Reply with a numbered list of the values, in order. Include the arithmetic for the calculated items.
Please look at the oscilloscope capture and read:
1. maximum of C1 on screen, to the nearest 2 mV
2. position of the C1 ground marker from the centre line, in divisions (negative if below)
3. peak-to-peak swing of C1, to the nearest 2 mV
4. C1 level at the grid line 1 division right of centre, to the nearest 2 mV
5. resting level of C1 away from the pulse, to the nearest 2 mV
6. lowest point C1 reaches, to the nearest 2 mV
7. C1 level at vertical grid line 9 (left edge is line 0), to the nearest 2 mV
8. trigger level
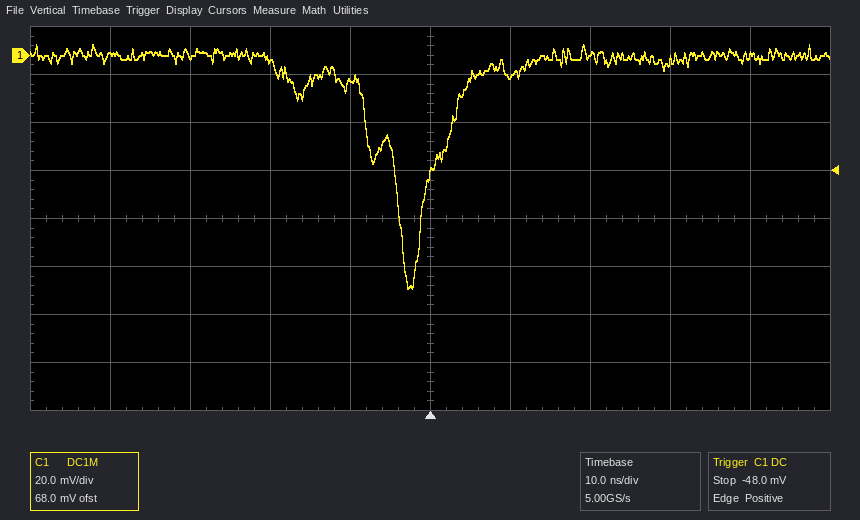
1. 4 mV
2. +3.4 div
3. 4 mV − (-98 mV) = 102 mV
4. -8 mV
5. 0 mV
6. -98 mV
7. 0 mV
8. -48.0 mV
